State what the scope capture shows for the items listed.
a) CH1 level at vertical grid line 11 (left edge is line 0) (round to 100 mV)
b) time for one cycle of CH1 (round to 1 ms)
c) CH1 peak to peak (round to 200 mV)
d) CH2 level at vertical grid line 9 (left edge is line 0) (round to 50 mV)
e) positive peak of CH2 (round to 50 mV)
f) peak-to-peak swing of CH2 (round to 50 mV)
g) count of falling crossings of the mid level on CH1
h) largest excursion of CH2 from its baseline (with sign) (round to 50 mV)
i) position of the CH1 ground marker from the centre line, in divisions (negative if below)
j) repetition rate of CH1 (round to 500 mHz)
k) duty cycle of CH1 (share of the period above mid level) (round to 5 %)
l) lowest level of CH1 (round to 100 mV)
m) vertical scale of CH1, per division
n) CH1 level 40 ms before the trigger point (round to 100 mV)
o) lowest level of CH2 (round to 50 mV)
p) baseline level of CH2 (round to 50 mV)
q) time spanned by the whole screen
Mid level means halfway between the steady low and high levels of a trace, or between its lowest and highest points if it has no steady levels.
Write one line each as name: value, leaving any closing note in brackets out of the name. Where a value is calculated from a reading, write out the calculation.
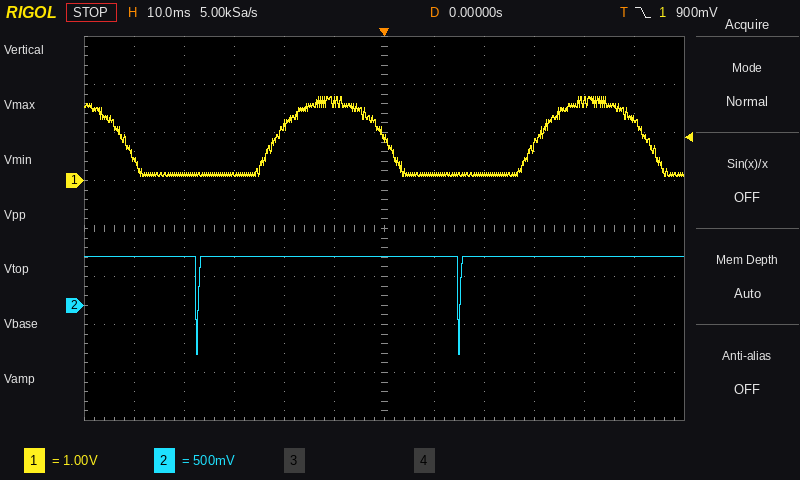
CH1 level at vertical grid line 11 (left edge is line 0): 1.3 V
time for one cycle of CH1: 52 ms
CH1 peak to peak: 1.6 V
CH2 level at vertical grid line 9 (left edge is line 0): 500 mV
positive peak of CH2: 500 mV
peak-to-peak swing of CH2: 500 mV − (-500 mV) = 1.00 V
count of falling crossings of the mid level on CH1: 3
largest excursion of CH2 from its baseline (with sign): -500 mV − (500 mV) = -1.00 V
position of the CH1 ground marker from the centre line, in divisions: +1.0 div
repetition rate of CH1: 1 / 52 ms ≈ 19.2 Hz, so 19.0 Hz to the nearest 500 mHz
duty cycle of CH1 (share of the period above mid level): 40 %
lowest level of CH1: 100 mV
vertical scale of CH1, per division: 1 V
CH1 level 40 ms before the trigger point: 100 mV
lowest level of CH2: -500 mV
baseline level of CH2: 500 mV
time spanned by the whole screen: 120 ms
